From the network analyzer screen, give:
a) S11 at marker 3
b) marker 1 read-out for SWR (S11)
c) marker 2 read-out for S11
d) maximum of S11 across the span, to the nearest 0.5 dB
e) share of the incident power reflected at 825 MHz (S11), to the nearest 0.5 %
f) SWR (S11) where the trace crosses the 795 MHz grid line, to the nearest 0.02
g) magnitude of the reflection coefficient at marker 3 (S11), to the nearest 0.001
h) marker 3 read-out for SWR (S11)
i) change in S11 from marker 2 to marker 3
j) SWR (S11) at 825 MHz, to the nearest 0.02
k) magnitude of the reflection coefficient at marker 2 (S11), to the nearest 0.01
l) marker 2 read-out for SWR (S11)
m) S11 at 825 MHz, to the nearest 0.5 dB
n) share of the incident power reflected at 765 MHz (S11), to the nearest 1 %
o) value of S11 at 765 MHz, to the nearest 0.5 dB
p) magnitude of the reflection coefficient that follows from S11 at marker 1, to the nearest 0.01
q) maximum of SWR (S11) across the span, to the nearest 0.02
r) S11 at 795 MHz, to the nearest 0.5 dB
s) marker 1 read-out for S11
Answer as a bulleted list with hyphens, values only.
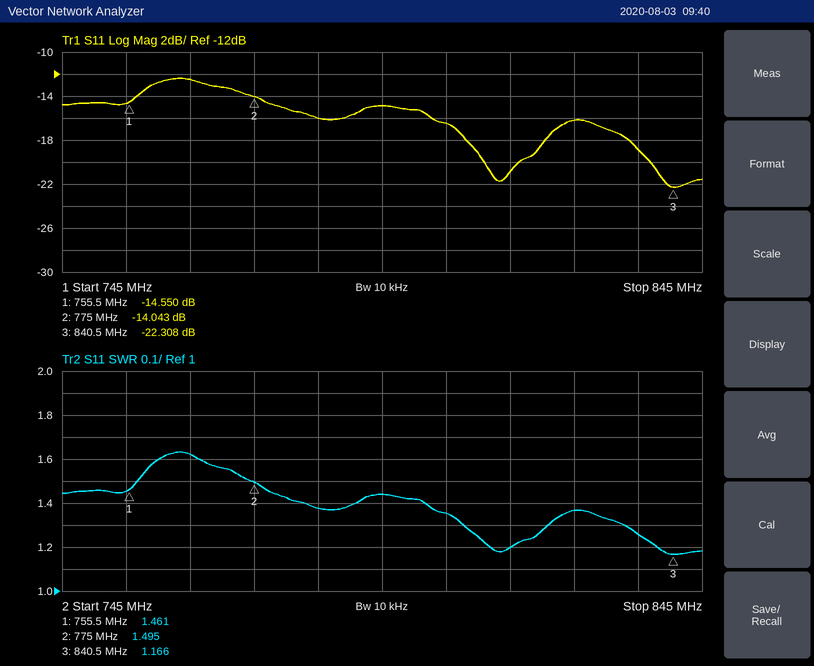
- -22.308 dB
- 1.461
- -14.043 dB
- -12.5 dB
- 2.5 %
- 1.44
- 0.077
- 1.166
- -8.265 dB
- 1.36
- 0.20
- 1.495
- -16.0 dB
- 6 %
- -12.5 dB
- 0.19
- 1.64
- -15.0 dB
- -14.550 dB
